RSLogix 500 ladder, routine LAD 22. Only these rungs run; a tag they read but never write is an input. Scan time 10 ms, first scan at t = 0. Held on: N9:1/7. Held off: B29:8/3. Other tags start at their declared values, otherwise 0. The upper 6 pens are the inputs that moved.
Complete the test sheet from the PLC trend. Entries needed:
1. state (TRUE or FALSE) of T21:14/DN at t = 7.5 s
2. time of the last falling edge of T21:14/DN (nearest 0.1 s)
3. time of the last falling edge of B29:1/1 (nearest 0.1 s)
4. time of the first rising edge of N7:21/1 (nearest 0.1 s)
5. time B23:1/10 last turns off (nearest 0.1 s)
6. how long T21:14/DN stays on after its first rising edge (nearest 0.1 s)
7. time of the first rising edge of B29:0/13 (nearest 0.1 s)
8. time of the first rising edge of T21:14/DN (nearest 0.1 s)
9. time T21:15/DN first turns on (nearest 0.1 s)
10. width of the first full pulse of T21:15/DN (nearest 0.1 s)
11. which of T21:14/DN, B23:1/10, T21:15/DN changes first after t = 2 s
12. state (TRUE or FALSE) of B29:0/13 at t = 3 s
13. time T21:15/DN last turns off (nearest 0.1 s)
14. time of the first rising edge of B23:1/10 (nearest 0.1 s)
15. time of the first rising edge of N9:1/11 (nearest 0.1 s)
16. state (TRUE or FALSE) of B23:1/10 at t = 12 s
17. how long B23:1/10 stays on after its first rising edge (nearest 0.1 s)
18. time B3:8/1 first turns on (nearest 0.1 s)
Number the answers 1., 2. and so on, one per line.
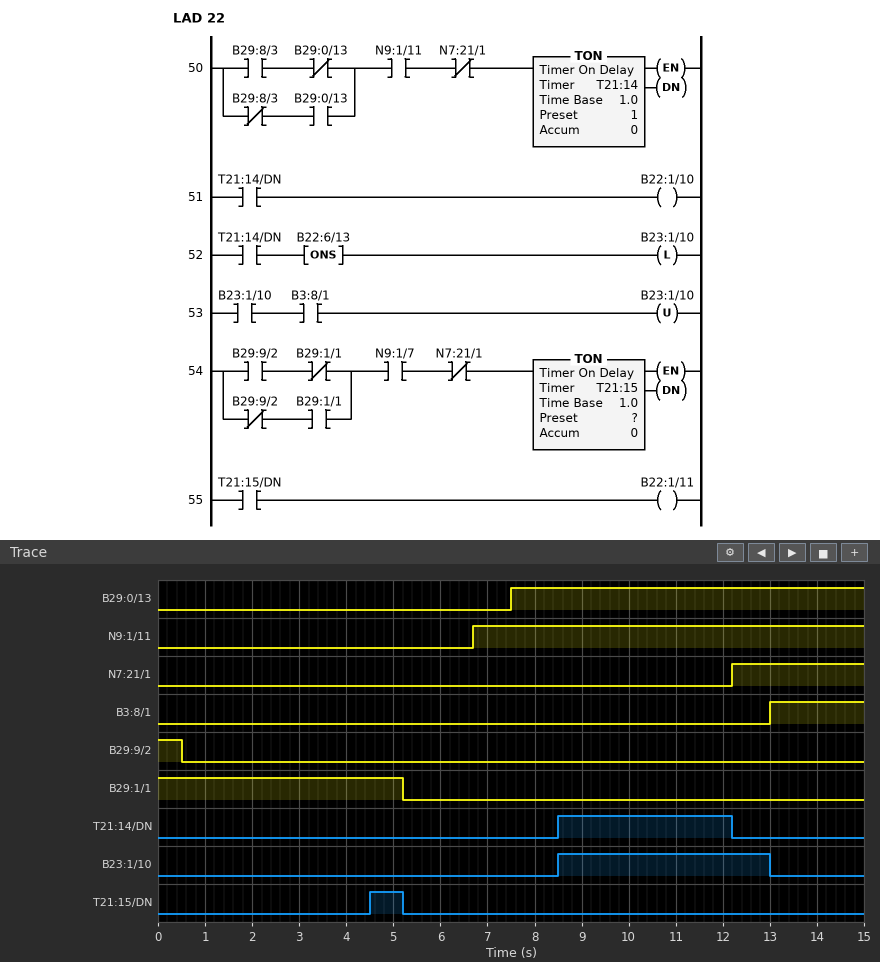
1. FALSE
2. 12.2 s
3. 5.2 s
4. 12.2 s
5. 13.0 s
6. 3.7 s
7. 7.5 s
8. 8.5 s
9. 4.5 s
10. 0.7 s
11. T21:15/DN
12. FALSE
13. 5.2 s
14. 8.5 s
15. 6.7 s
16. TRUE
17. 4.5 s
18. 13.0 s
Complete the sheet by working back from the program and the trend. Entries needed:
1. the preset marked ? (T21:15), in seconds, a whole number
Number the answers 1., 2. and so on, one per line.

1. 4 s
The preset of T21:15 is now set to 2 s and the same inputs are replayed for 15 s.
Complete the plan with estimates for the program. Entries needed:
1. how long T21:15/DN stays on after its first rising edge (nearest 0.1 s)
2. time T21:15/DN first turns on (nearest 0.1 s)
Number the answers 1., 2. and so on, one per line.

1. 2.7 s
2. 2.5 s
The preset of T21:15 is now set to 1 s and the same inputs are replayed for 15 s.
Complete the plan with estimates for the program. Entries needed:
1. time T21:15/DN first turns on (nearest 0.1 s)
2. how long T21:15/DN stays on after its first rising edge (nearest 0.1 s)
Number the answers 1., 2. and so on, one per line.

1. 1.5 s
2. 3.7 s
